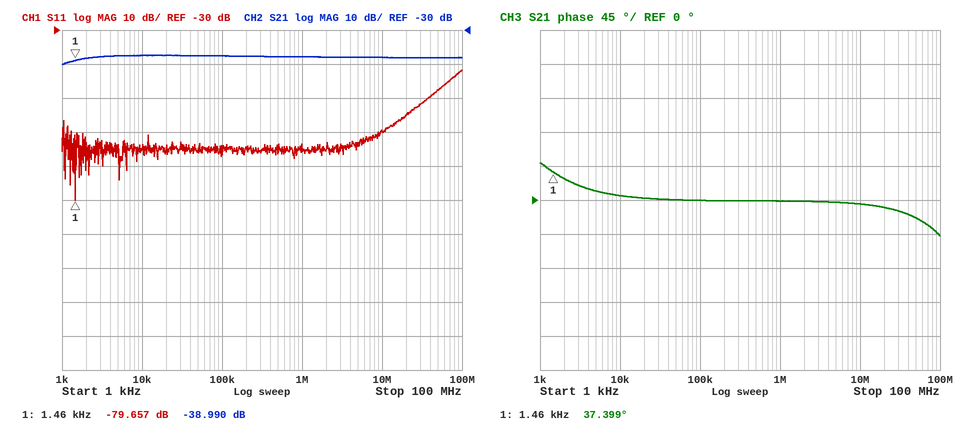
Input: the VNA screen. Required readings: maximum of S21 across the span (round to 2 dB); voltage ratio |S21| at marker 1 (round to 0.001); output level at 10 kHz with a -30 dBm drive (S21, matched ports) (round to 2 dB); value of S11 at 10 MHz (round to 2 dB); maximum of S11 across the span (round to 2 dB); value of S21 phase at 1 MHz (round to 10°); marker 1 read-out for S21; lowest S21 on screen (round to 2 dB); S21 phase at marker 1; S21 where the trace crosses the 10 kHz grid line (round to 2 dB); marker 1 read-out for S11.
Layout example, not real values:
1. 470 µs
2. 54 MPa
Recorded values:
1. -38 dB
2. 0.011
3. -68 dBm
4. -60 dB
5. -42 dB
6. 0°
7. -38.990 dB
8. -40 dB
9. 37.399°
10. -38 dB
11. -79.657 dB
